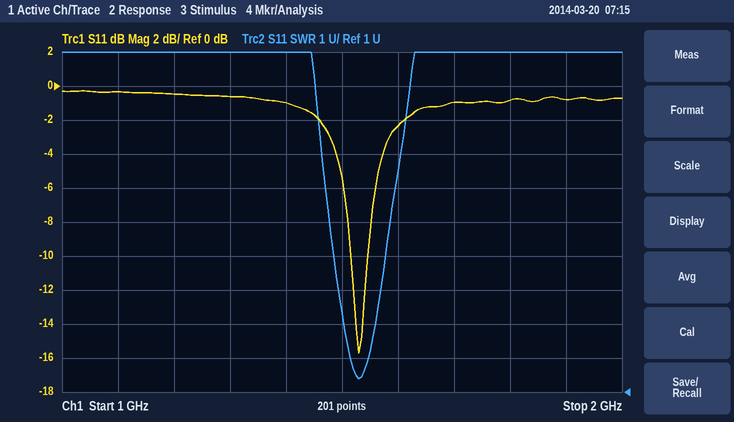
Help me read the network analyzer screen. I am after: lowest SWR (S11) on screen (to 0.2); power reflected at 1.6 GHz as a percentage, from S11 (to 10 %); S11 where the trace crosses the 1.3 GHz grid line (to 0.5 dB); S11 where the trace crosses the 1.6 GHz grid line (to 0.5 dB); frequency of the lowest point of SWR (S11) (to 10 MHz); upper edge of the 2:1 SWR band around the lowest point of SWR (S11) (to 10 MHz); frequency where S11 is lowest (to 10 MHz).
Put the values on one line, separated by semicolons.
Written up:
1.4; 60 %; -0.5 dB; -2.5 dB; 1.53 GHz; 1.55 GHz; 1.53 GHz
